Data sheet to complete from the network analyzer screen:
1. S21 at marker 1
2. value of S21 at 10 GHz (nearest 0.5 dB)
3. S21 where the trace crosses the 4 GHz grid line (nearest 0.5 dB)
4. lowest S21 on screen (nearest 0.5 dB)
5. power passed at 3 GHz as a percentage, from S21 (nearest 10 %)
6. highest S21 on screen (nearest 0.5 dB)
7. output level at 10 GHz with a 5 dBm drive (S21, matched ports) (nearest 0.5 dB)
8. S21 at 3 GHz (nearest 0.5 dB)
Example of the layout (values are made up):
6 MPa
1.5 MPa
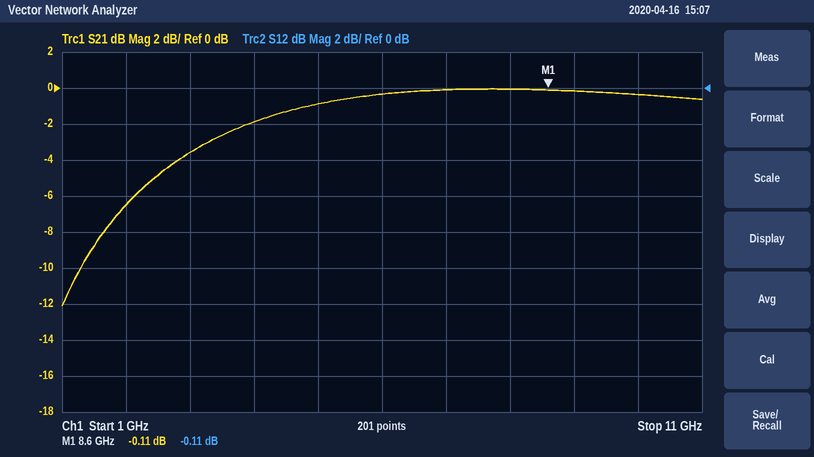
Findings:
-0.11 dB
-0.5 dB
-2.0 dB
-12.0 dB
40 %
0.0 dB
4.5 dBm
-3.5 dB
